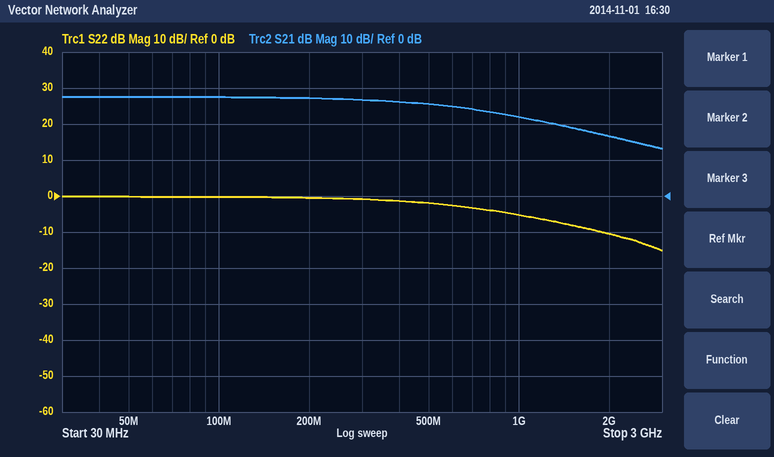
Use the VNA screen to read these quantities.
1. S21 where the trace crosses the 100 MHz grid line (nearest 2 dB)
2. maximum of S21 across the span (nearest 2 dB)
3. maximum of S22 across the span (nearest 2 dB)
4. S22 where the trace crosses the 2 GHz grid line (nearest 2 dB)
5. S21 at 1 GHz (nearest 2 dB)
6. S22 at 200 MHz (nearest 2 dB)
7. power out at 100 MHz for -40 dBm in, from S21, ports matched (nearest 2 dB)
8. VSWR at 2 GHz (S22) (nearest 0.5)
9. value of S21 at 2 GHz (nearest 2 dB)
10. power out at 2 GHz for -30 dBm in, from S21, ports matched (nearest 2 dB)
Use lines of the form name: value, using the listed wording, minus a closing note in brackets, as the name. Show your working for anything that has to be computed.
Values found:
S21 where the trace crosses the 100 MHz grid line: 28 dB
maximum of S21 across the span: 28 dB
maximum of S22 across the span: 0 dB
S22 where the trace crosses the 2 GHz grid line: -10 dB
S21 at 1 GHz: 22 dB
S22 at 200 MHz: 0 dB
power out at 100 MHz for -40 dBm in, from S21, ports matched: -40 dBm + (28 dB) = -12 dBm
VSWR at 2 GHz (S22): |Γ| = 10^(-10/20) = 0.3162; VSWR = (1 + 0.3162)/(1 − 0.3162) ≈ 1.92, so 2.0 to the nearest 0.5
value of S21 at 2 GHz: 16 dB
power out at 2 GHz for -30 dBm in, from S21, ports matched: -30 dBm + (16 dB) = -14 dBm
